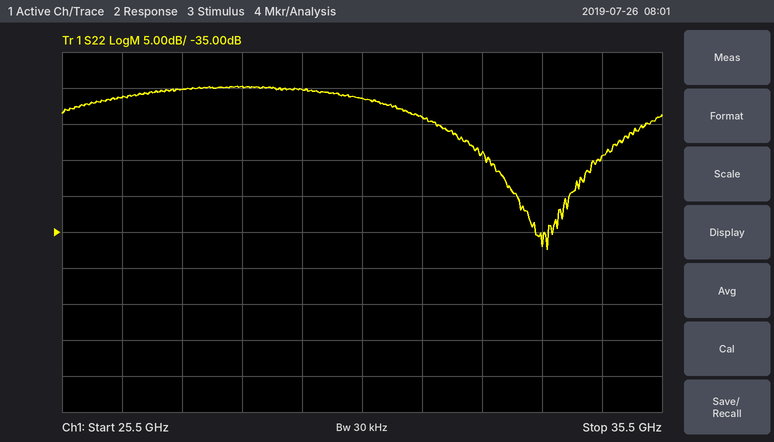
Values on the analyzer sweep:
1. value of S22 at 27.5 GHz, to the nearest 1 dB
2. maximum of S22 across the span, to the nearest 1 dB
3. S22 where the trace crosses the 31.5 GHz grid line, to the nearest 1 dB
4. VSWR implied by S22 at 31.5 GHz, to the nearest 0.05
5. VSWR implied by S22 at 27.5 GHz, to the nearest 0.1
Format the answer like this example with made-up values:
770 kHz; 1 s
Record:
-15 dB; -15 dB; -19 dB; 1.25; 1.4
